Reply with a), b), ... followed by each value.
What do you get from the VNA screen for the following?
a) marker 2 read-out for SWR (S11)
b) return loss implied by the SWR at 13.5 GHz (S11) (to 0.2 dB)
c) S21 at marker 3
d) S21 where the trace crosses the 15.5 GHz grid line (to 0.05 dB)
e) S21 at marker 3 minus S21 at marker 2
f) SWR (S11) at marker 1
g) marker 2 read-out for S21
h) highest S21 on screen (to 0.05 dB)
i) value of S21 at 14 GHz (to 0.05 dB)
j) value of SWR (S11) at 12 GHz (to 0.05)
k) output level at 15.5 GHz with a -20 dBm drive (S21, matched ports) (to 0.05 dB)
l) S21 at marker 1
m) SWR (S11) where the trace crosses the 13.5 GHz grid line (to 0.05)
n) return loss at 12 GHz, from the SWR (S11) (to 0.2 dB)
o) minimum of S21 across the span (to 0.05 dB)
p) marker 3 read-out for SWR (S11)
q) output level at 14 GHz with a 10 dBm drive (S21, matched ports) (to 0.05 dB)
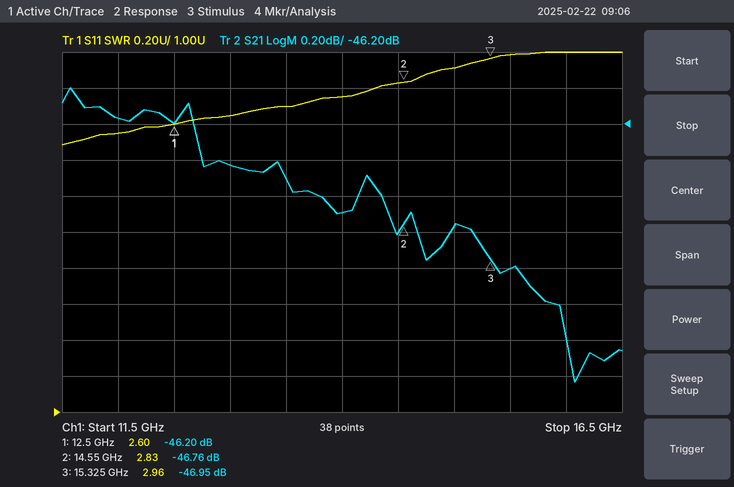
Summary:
a) 2.83
b) 6.8 dB
c) -46.95 dB
d) -47.00 dB
e) -0.19 dB
f) 2.60
g) -46.76 dB
h) -46.00 dB
i) -46.70 dB
j) 2.55
k) -67.00 dBm
l) -46.20 dB
m) 2.70
n) 7.2 dB
o) -47.65 dB
p) 2.96
q) -36.70 dBm
